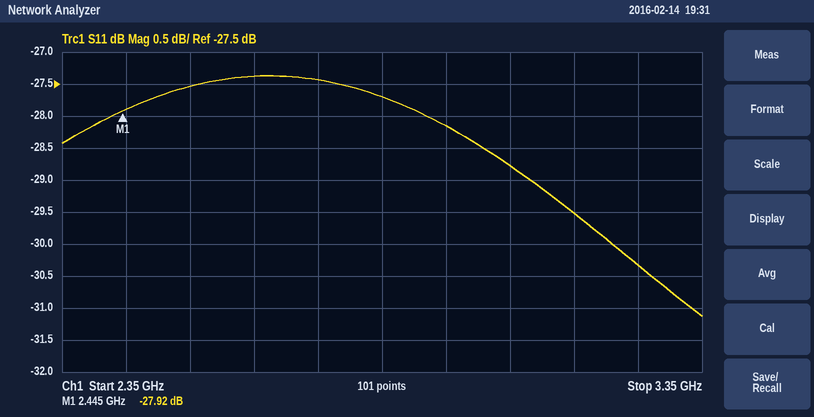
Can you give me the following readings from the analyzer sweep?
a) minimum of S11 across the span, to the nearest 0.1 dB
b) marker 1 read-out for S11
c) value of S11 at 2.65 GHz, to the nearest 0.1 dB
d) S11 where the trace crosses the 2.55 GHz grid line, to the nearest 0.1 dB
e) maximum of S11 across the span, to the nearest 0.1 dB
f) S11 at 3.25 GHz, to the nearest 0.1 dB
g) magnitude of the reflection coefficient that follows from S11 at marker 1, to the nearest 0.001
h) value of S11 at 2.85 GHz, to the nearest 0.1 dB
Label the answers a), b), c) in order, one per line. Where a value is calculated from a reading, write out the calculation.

a) -31.1 dB
b) -27.92 dB
c) -27.4 dB
d) -27.5 dB
e) -27.4 dB
f) -30.3 dB
g) 10^(-27.92/20) ≈ 0.040
h) -27.7 dB
